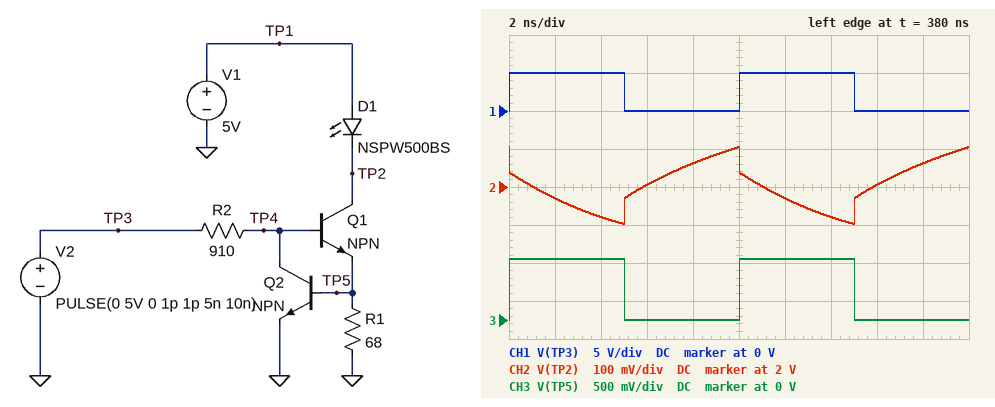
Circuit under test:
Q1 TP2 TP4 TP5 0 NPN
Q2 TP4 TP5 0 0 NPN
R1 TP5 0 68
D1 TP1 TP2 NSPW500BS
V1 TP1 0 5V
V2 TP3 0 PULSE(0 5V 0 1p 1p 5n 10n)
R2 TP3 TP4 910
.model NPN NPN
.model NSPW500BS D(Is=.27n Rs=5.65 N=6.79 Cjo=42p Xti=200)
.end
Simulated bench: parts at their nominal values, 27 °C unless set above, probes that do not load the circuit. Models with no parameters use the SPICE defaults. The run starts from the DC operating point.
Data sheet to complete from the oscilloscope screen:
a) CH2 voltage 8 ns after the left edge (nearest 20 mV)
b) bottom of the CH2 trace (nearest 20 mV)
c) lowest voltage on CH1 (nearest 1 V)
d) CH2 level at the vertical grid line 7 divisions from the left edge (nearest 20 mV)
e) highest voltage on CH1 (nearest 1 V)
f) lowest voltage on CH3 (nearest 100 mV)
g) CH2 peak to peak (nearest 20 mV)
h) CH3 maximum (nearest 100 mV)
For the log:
2.06 V
1.90 V
0 V
1.92 V
5 V
0 V
200 mV
800 mV
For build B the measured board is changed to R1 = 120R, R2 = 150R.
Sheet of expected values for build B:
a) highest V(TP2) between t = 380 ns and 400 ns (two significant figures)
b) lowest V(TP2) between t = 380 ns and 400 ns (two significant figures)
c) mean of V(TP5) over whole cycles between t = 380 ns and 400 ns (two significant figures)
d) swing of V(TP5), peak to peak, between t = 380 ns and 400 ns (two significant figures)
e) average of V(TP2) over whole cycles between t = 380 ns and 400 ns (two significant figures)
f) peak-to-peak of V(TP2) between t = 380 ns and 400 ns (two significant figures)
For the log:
2.2 V
2.0 V
430 mV
850 mV
2.1 V
130 mV
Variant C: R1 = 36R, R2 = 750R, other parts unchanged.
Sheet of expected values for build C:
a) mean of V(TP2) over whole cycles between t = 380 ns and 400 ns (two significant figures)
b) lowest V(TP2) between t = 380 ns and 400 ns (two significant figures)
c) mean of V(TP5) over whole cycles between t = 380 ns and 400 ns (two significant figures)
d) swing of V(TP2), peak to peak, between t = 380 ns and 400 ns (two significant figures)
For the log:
1.9 V
1.7 V
410 mV
350 mV
